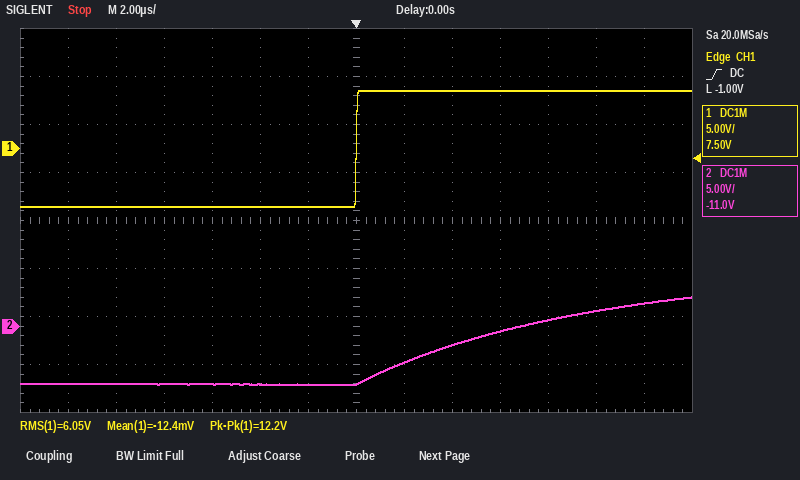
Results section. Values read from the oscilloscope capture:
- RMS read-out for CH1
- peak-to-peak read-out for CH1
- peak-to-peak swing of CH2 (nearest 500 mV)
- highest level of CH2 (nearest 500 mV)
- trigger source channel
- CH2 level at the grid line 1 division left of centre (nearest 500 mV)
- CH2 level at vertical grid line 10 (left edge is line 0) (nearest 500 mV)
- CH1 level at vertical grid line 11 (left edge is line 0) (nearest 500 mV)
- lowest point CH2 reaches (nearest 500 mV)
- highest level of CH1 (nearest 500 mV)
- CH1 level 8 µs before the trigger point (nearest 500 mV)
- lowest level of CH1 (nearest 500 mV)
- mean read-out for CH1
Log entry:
6.05 V
12.2 V
9.0 V
3.0 V
CH1
-6.0 V
-500 mV
6.0 V
-6.0 V
6.0 V
-6.0 V
-6.0 V
-12.4 mV
